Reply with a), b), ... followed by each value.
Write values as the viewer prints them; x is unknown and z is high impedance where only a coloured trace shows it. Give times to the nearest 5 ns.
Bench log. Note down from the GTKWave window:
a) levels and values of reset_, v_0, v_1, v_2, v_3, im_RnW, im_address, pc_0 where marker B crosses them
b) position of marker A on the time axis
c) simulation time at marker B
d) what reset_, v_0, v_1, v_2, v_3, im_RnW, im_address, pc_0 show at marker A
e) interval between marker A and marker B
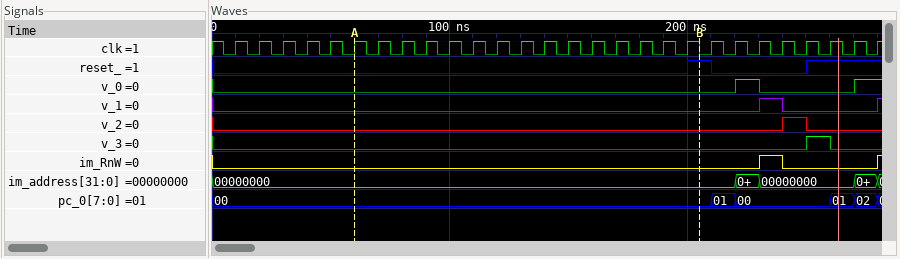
a) reset_=1, v_0=0, v_1=0, v_2=0, v_3=0, im_RnW=0, im_address=00000000, pc_0=00
b) 60 ns
c) 205 ns
d) reset_=0, v_0=0, v_1=0, v_2=0, v_3=0, im_RnW=0, im_address=00000000, pc_0=00
e) 145 ns
